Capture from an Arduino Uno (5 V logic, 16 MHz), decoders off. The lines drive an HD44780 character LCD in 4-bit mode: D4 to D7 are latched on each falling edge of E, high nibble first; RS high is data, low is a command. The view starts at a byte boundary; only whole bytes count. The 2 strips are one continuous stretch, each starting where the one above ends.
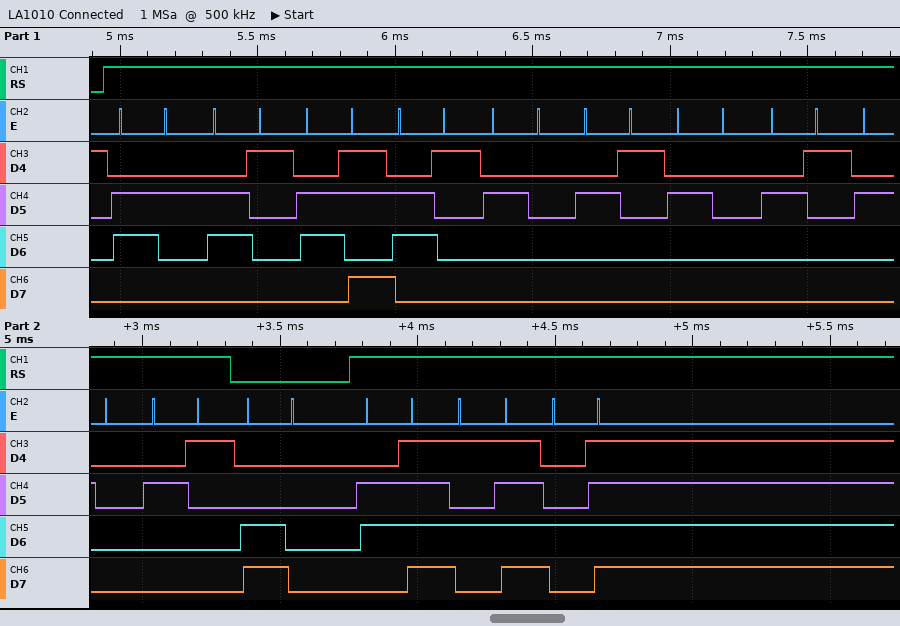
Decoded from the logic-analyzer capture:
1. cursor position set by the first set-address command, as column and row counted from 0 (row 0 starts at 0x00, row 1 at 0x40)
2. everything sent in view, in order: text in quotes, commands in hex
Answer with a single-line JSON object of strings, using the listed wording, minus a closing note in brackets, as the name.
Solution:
{"cursor position set by the first set-address command, as column and row counted from 0": "column 0, row 1", "everything sent in view, in order: text in quotes, commands in hex": "\"baka ! ! !\" 0xC0 \"o_O\""}
